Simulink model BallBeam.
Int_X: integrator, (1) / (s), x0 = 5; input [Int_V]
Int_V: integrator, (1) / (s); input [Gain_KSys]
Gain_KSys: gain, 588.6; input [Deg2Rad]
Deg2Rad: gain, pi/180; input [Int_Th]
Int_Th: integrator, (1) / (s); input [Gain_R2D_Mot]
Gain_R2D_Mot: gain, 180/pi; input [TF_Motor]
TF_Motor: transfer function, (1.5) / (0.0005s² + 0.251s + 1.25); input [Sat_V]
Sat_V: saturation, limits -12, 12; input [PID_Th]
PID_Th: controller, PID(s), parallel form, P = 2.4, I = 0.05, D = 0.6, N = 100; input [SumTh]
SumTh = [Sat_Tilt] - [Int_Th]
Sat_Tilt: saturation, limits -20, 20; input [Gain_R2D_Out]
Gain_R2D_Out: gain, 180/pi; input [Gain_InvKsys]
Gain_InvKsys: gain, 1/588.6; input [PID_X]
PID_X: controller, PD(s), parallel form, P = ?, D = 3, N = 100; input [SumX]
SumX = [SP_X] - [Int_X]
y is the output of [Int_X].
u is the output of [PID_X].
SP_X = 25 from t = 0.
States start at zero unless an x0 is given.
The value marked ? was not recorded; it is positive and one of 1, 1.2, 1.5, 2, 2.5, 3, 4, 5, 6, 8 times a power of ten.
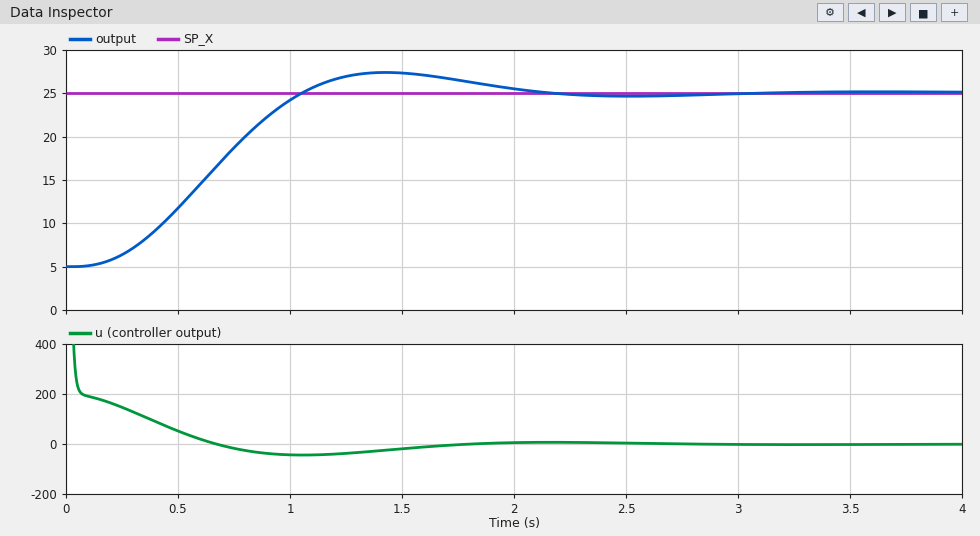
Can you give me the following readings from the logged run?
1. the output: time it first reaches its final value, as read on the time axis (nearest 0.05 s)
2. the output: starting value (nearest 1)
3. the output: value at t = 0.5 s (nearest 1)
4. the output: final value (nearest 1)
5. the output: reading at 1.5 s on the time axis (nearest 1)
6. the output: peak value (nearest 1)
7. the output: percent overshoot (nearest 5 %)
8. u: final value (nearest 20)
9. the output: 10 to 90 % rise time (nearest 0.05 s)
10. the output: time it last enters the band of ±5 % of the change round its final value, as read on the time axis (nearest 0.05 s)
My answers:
1.05 s
5
12
25
27
27
10 %
0
0.65 s
1.85 s
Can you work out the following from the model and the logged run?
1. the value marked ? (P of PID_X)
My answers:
10
